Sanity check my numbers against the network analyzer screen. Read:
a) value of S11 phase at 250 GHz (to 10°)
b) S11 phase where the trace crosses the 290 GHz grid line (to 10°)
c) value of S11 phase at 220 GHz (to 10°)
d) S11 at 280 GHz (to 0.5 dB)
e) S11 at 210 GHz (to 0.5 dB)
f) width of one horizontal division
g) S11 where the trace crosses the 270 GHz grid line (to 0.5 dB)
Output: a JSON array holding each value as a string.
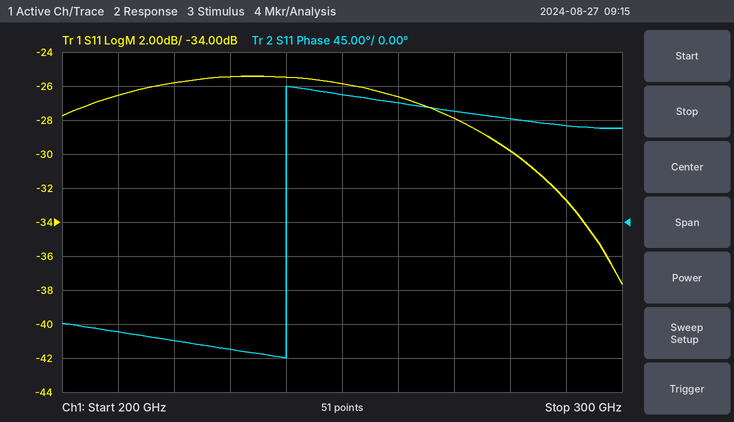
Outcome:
["170°", "130°", "-160°", "-30.0 dB", "-26.5 dB", "10 GHz", "-28.0 dB"]
